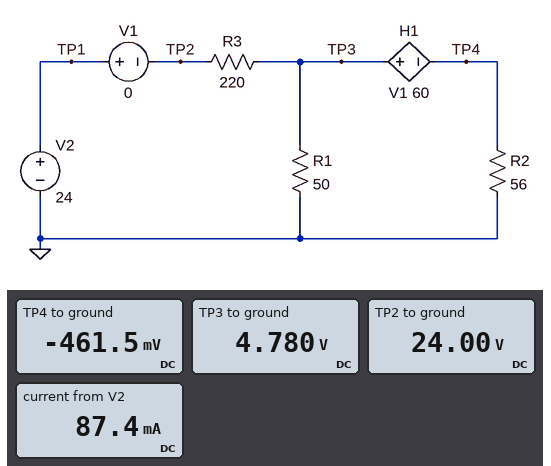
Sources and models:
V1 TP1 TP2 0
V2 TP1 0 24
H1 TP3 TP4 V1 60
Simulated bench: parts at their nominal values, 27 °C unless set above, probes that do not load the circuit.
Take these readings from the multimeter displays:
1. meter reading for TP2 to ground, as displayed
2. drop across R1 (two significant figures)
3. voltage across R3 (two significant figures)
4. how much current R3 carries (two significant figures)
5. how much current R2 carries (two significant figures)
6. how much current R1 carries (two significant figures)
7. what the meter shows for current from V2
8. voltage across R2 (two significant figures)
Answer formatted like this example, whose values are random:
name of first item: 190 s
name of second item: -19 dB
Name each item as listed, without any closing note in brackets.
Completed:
meter reading for TP2 to ground, as displayed: 24.00 V
drop across R1: 4.8 V
voltage across R3: 19 V
how much current R3 carries: 87 mA
how much current R2 carries: 8.2 mA
how much current R1 carries: 96 mA
what the meter shows for current from V2: 87.4 mA
voltage across R2: 460 mV
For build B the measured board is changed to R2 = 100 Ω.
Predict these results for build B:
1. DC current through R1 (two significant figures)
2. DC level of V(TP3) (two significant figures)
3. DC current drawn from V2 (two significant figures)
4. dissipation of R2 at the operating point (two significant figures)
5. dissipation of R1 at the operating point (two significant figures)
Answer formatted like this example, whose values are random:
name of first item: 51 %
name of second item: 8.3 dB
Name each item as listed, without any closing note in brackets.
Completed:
DC current through R1: 94 mA
DC level of V(TP3): 4.7 V
DC current drawn from V2: 88 mA
dissipation of R2 at the operating point: 3.4 mW
dissipation of R1 at the operating point: 440 mW
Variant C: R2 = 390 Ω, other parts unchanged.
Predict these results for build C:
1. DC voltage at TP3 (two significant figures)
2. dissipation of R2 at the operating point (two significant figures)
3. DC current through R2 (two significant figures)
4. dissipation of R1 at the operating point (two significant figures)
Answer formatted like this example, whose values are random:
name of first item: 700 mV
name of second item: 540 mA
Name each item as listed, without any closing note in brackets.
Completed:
DC voltage at TP3: 4.5 V
dissipation of R2 at the operating point: 1.6 mW
DC current through R2: 2.0 mA
dissipation of R1 at the operating point: 410 mW
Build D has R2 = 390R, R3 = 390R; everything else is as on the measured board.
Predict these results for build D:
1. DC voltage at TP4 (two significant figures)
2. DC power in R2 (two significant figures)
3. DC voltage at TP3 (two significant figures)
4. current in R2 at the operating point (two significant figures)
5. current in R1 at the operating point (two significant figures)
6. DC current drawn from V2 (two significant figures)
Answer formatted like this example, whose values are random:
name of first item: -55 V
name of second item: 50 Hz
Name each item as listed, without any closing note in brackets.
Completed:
DC voltage at TP4: -480 mV
DC power in R2: 600 µW
DC voltage at TP3: 2.8 V
current in R2 at the operating point: 1.2 mA
current in R1 at the operating point: 56 mA
DC current drawn from V2: 54 mA
